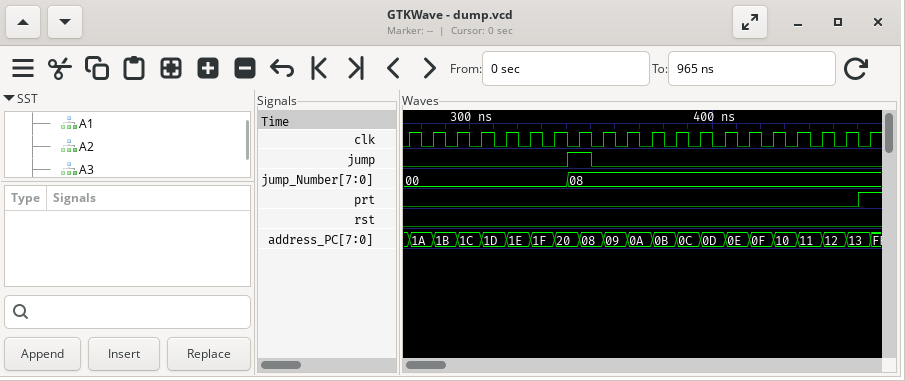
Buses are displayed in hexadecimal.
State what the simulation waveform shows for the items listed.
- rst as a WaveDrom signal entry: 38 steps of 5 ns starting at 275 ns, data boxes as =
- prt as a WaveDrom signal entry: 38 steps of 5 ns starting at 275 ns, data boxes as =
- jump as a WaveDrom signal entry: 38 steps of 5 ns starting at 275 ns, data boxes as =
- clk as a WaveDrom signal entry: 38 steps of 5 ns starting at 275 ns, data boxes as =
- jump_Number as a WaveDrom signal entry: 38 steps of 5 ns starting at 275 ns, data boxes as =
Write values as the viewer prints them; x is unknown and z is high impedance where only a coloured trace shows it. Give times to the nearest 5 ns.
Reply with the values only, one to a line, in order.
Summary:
{name: 'rst', wave: '0.....................................'}
{name: 'prt', wave: '0....................................1'}
{name: 'jump', wave: '0............1.0......................'}
{name: 'clk', wave: '10101010101010101010101010101010101010'}
{name: 'jump_Number', wave: '=............=........................', data: '00 08'}
